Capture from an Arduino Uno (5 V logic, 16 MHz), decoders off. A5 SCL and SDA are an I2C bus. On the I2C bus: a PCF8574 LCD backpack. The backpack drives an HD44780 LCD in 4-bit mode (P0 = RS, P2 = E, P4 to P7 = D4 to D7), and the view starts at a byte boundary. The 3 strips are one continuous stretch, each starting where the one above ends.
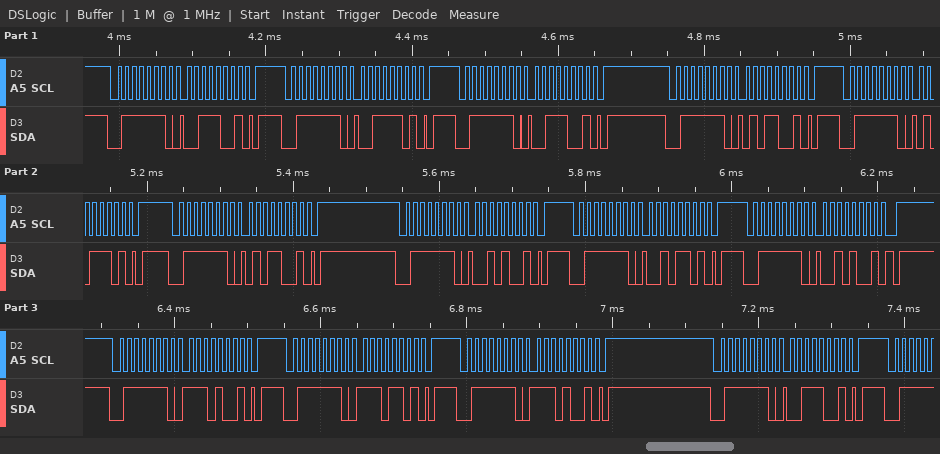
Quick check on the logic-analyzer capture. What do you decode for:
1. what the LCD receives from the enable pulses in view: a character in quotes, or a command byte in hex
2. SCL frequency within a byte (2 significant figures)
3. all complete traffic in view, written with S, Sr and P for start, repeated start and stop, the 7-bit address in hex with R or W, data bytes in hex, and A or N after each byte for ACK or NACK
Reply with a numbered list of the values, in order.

1. '5' '.'
2. 100 kHz
3. S 3FW A 39 A P S 3FW A 3D A P S 3FW A 39 A P S 3FW A 59 A P S 3FW A 5D A P S 3FW A 59 A P S 3FW A 29 A P S 3FW A 2D A P S 3FW A 29 A P S 3FW A E9 A P S 3FW A ED A P S 3FW A E9 A P S 3FW A 39 A P
